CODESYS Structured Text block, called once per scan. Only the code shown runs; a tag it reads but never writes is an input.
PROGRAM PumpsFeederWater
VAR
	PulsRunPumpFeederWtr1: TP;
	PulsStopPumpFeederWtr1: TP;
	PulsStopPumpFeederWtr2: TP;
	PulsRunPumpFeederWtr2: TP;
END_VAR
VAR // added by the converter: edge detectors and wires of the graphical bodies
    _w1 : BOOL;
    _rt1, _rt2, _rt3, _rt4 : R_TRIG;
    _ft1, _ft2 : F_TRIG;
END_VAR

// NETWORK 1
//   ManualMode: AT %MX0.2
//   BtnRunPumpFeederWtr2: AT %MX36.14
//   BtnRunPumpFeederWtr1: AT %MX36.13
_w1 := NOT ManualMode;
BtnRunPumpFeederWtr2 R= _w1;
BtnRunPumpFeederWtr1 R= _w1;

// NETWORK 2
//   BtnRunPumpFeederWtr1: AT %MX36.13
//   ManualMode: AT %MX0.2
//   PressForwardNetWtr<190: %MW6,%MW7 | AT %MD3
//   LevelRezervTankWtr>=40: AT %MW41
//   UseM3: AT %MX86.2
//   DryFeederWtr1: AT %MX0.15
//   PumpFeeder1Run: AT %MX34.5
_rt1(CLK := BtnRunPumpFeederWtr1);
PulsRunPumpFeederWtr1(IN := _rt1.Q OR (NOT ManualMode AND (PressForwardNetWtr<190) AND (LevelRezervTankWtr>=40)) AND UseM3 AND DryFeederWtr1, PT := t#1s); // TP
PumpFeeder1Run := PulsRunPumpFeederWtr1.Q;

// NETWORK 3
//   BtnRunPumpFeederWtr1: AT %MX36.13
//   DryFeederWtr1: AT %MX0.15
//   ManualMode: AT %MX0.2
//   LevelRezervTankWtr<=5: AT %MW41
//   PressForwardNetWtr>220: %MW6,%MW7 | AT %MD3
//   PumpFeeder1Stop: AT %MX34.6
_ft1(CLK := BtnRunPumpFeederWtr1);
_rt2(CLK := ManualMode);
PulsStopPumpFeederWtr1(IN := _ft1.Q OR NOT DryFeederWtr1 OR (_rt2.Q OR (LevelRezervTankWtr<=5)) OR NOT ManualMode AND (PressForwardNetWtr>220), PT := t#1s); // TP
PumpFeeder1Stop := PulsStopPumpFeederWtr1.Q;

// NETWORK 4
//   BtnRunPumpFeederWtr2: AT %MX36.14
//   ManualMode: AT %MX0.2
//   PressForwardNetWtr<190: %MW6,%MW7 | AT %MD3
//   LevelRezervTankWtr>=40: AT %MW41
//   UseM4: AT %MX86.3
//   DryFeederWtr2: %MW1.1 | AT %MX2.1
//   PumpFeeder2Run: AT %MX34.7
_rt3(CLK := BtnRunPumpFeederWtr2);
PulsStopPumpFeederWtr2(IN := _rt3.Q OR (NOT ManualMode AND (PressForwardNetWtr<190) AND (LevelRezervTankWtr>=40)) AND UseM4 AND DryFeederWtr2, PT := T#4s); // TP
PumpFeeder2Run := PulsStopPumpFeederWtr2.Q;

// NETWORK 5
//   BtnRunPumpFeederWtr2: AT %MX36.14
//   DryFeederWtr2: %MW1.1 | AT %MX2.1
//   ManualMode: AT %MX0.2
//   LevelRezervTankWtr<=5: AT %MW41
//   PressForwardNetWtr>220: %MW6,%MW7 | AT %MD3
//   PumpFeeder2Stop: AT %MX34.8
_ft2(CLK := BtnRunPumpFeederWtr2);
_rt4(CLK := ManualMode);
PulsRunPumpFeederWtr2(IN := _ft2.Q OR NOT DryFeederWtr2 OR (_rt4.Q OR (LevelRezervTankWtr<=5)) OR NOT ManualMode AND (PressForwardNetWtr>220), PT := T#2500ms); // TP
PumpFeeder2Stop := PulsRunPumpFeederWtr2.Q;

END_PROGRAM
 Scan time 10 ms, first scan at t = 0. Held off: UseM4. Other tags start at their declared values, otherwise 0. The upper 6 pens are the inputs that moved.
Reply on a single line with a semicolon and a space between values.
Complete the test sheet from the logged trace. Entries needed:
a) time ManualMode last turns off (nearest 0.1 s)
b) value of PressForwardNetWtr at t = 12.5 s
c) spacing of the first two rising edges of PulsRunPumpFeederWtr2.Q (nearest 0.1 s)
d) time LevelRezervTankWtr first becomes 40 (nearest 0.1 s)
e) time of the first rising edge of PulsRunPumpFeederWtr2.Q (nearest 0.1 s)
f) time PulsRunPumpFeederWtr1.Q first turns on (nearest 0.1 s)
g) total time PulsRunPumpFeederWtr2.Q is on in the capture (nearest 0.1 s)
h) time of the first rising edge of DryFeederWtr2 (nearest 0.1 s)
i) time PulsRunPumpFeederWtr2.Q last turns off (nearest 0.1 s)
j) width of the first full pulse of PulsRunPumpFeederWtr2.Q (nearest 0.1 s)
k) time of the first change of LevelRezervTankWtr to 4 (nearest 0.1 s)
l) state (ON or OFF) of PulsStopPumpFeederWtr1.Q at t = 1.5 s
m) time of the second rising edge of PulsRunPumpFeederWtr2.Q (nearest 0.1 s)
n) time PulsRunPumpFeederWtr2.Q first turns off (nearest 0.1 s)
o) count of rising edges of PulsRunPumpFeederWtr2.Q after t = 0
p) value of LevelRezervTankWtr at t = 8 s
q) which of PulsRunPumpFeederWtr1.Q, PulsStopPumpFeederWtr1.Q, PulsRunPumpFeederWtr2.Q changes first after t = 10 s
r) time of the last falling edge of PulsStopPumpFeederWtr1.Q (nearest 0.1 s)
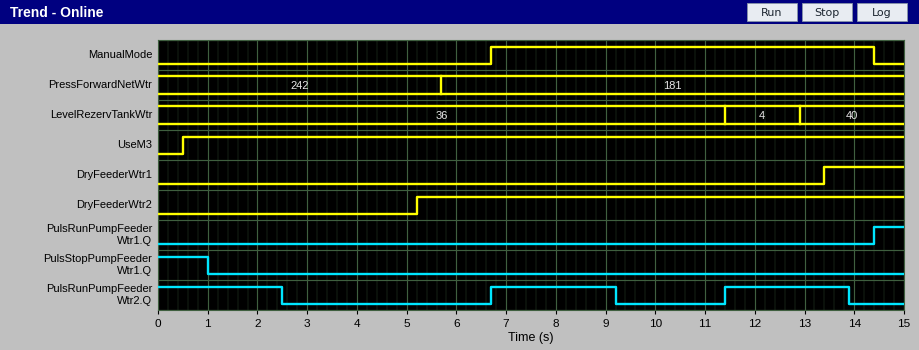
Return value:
14.4 s; 181; 4.7 s; 12.9 s; 6.7 s; 14.4 s; 7.5 s; 5.2 s; 13.9 s; 2.5 s; 11.4 s; OFF; 11.4 s; 2.5 s; 2; 36; PulsRunPumpFeederWtr2.Q; 1.0 s
